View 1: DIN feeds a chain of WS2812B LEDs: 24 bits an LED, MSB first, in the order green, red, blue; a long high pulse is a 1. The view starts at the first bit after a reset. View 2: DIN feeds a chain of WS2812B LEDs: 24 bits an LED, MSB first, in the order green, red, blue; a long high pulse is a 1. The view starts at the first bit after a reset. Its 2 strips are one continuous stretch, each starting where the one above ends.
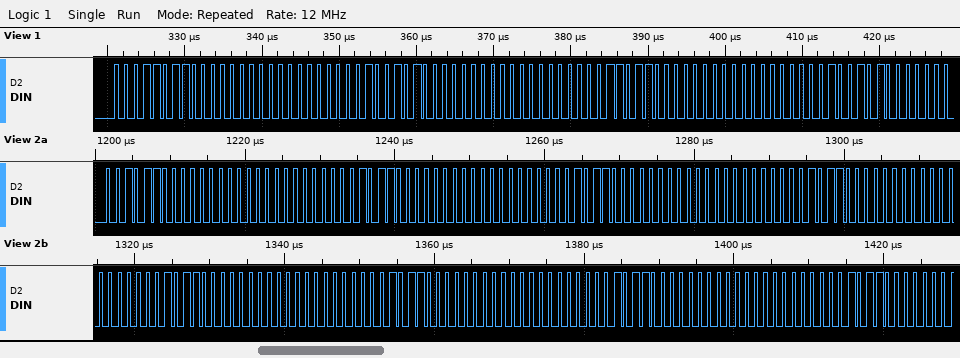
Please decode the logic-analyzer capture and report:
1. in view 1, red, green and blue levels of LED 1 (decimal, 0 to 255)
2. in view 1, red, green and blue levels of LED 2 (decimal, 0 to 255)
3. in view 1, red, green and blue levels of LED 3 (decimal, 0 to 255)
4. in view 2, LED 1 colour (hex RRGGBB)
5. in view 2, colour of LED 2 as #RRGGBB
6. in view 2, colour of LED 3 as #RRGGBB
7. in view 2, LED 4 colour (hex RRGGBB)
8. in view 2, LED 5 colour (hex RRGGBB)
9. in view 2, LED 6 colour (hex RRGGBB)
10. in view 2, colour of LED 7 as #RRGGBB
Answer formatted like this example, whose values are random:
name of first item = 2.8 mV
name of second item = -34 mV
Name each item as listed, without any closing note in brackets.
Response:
in view 1, red, green and blue levels of LED 1 = 0, 27, 0
in view 1, red, green and blue levels of LED 2 = 0, 37, 0
in view 1, red, green and blue levels of LED 3 = 0, 27, 0
in view 2, LED 1 colour = #002C00
in view 2, colour of LED 2 as #RRGGBB = #001600
in view 2, colour of LED 3 as #RRGGBB = #002C00
in view 2, LED 4 colour = #001600
in view 2, LED 5 colour = #002C00
in view 2, LED 6 colour = #002C00
in view 2, colour of LED 7 as #RRGGBB = #002C00
